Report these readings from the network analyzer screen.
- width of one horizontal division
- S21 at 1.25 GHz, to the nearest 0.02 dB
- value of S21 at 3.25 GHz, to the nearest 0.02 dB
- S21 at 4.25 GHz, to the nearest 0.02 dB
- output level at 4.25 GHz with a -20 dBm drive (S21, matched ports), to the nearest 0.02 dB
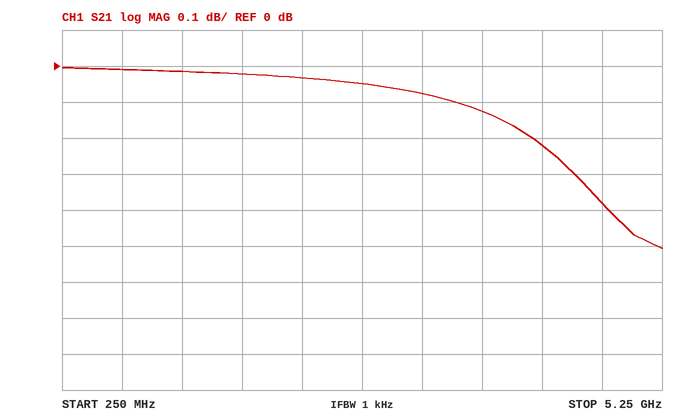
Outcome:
500 MHz
-0.02 dB
-0.08 dB
-0.22 dB
-20.22 dBm
